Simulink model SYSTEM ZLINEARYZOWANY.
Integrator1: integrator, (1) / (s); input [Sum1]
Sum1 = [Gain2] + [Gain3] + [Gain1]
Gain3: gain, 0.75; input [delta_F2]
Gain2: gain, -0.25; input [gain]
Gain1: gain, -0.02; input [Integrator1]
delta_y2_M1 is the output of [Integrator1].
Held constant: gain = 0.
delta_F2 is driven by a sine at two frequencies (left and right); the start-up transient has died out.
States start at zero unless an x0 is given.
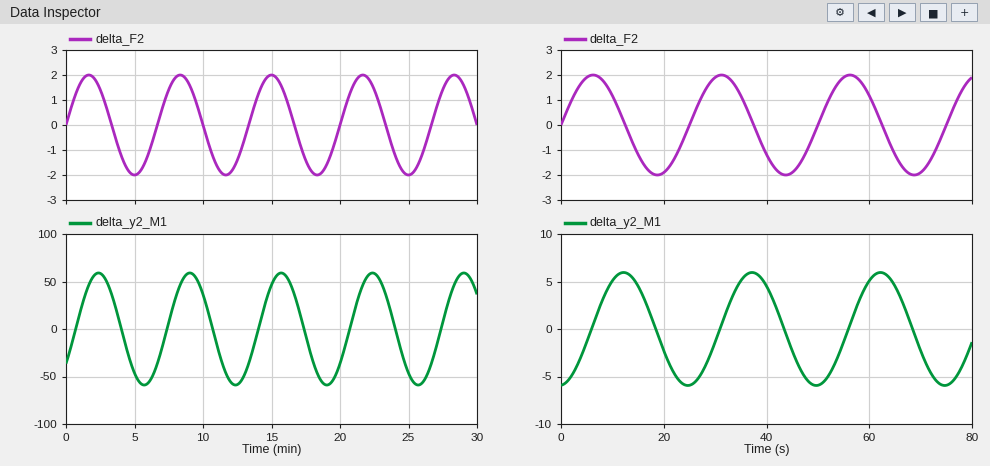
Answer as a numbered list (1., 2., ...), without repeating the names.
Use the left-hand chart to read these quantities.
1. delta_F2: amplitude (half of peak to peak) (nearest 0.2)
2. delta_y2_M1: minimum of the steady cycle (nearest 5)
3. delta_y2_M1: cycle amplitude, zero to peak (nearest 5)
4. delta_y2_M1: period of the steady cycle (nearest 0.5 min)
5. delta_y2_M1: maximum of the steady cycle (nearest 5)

1. 2.0
2. -60
3. 60
4. 6.5 min
5. 60
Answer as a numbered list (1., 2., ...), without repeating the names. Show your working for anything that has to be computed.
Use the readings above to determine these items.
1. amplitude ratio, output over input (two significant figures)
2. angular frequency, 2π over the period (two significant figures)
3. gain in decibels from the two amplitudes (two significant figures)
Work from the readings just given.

1. 60 / 2 = 30
2. 2π / 6.5 = 0.97 rad/min
3. 20 log10(60 / 2) = 30 dB
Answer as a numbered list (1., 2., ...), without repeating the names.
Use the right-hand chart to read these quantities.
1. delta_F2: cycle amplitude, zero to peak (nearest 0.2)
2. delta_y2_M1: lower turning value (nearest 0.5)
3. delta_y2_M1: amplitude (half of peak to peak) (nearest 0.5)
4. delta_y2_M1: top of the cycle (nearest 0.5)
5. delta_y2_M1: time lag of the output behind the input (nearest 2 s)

1. 2.0
2. -6.0
3. 6.0
4. 6.0
5. 6 s
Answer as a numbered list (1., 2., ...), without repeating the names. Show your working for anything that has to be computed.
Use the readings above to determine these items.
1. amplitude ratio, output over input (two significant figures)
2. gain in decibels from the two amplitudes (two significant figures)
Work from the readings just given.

1. 6 / 2 = 3.0
2. 20 log10(6 / 2) = 9.5 dB
